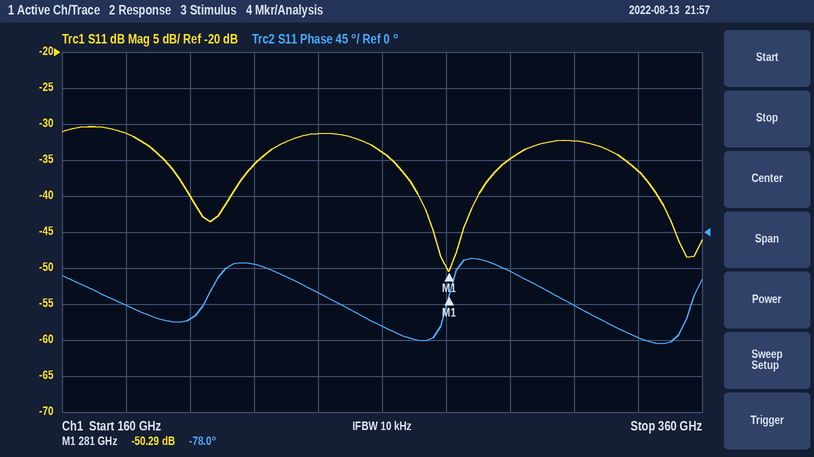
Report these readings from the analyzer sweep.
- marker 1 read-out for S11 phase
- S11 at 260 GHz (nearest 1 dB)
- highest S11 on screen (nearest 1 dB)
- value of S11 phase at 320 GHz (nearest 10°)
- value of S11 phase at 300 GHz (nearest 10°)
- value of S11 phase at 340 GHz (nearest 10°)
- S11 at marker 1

-78.0°
-34 dB
-30 dB
-90°
-50°
-130°
-50.29 dB
